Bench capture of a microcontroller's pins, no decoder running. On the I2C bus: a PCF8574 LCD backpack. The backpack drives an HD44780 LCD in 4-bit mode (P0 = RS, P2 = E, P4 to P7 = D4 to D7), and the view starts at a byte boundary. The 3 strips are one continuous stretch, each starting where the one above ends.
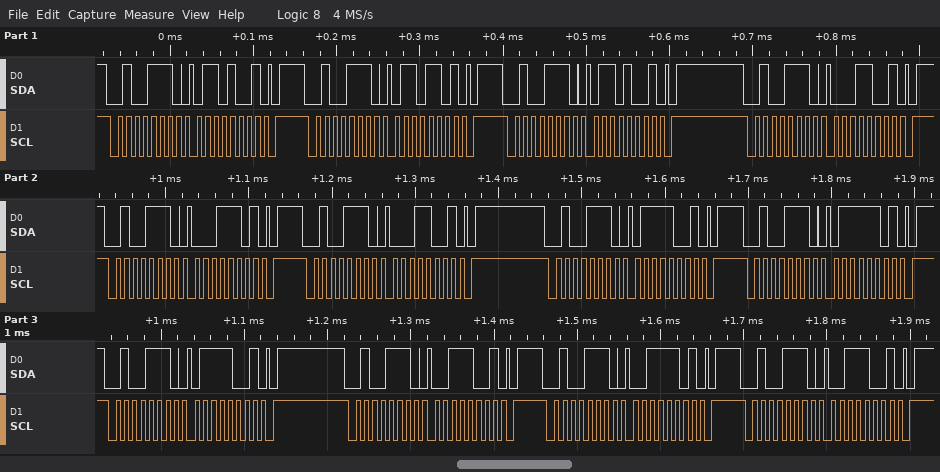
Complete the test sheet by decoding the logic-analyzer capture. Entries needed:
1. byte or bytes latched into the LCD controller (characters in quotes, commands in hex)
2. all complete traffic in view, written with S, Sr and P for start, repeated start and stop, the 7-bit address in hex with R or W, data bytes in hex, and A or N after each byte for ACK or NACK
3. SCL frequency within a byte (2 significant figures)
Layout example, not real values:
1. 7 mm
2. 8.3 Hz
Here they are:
1. 'a' 's'
2. S 27W A 69 A P S 27W A 6D A P S 27W A 69 A P S 27W A 19 A P S 27W A 1D A P S 27W A 19 A P S 27W A 79 A P S 27W A 7D A P S 27W A 79 A P S 27W A 39 A P S 27W A 3D A P S 27W A 39 A P
3. 100 kHz
